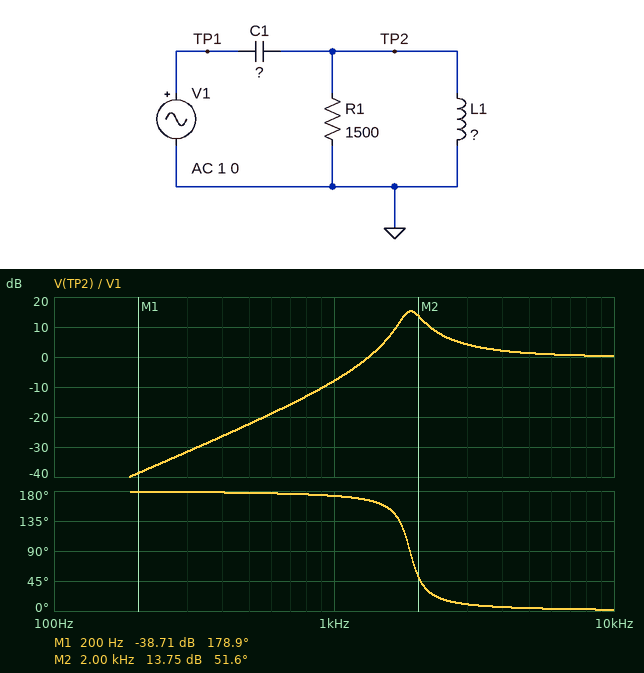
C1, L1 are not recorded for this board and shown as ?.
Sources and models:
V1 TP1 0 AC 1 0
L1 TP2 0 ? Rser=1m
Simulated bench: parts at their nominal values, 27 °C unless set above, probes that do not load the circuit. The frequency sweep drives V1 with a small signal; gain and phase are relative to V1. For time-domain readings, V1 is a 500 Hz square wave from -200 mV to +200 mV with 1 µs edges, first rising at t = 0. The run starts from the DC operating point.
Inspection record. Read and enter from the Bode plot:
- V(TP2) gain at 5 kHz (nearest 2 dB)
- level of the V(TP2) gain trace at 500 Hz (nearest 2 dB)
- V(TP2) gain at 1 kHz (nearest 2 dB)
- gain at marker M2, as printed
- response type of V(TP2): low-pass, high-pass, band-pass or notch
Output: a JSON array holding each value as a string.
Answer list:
["2 dB", "-22 dB", "-8 dB", "13.75 dB", "high-pass"]
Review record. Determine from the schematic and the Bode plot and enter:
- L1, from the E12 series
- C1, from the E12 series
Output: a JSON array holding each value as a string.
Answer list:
["22 mH", "330 nF"]
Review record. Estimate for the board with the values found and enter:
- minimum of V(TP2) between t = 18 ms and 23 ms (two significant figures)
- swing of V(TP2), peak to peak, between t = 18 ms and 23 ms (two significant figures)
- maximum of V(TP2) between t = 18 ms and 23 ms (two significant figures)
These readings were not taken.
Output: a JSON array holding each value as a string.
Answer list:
["-300 mV", "600 mV", "300 mV"]
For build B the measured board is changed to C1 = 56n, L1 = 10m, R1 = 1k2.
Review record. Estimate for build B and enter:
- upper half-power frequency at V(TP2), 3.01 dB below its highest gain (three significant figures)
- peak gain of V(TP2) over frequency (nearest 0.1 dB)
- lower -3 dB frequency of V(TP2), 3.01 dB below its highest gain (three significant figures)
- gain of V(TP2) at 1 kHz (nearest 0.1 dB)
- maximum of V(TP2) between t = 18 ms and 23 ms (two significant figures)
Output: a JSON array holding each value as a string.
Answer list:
["8.75 kHz", "9.2 dB", "5.93 kHz", "-32.9 dB", "400 mV"]
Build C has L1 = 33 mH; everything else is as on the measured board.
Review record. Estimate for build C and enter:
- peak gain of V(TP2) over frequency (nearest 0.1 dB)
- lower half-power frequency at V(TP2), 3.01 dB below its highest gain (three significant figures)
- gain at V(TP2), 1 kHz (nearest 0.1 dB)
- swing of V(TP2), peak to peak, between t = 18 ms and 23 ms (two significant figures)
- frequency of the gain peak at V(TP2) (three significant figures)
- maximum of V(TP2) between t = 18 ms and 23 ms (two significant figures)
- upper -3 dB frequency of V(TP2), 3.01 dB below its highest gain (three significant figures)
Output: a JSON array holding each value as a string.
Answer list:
["13.6 dB", "1.40 kHz", "-2.7 dB", "1.2 V", "1.54 kHz", "620 mV", "1.74 kHz"]
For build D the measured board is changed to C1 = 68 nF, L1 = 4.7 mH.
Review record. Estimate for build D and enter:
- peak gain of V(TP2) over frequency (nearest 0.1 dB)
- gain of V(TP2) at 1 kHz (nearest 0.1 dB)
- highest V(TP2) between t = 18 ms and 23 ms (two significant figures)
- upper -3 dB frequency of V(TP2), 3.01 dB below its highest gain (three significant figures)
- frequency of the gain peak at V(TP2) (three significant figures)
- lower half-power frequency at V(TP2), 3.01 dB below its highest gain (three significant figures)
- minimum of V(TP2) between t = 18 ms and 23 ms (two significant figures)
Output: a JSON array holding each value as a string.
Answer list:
["15.2 dB", "-37.9 dB", "400 mV", "9.89 kHz", "8.97 kHz", "8.27 kHz", "-400 mV"]
